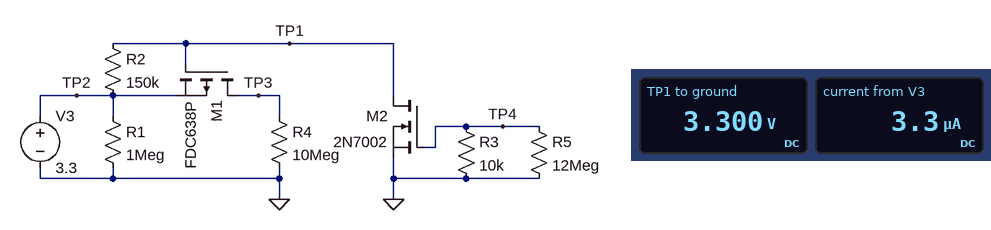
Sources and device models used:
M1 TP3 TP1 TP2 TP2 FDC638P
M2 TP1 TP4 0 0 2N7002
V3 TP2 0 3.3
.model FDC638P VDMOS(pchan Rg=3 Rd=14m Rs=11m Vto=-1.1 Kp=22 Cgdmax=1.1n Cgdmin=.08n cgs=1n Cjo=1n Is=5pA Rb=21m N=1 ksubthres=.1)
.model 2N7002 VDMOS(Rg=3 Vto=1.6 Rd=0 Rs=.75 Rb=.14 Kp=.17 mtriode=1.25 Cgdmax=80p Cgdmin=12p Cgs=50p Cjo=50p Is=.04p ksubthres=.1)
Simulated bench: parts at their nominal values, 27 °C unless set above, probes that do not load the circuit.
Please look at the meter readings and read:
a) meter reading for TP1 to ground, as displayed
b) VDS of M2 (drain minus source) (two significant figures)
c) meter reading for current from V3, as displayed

3.300 V
3.3 V
3.3 µA
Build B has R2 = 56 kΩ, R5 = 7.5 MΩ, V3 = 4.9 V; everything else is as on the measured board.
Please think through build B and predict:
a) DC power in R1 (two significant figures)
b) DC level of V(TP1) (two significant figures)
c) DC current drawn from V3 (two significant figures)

24 µW
4.9 V
4.9 µA
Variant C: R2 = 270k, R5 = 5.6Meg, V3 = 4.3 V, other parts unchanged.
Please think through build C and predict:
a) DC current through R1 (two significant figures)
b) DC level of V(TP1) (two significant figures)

4.3 µA
4.3 V
